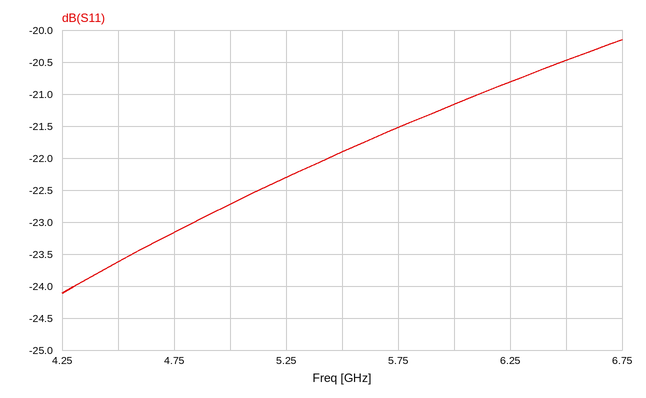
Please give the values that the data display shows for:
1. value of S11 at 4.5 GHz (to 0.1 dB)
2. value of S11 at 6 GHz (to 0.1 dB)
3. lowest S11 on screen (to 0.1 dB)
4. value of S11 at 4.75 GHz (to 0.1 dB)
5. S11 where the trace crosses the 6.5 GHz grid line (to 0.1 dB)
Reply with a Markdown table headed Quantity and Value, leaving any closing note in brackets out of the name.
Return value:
| Quantity | Value |
|---|---|
| value of S11 at 4.5 GHz | -23.6 dB |
| value of S11 at 6 GHz | -21.2 dB |
| lowest S11 on screen | -24.1 dB |
| value of S11 at 4.75 GHz | -23.2 dB |
| S11 where the trace crosses the 6.5 GHz grid line | -20.5 dB |
